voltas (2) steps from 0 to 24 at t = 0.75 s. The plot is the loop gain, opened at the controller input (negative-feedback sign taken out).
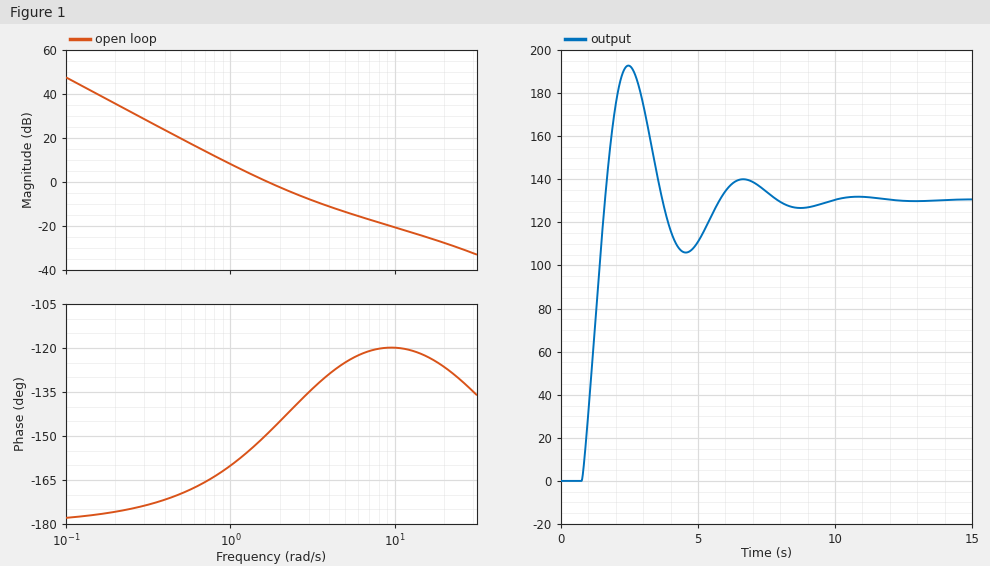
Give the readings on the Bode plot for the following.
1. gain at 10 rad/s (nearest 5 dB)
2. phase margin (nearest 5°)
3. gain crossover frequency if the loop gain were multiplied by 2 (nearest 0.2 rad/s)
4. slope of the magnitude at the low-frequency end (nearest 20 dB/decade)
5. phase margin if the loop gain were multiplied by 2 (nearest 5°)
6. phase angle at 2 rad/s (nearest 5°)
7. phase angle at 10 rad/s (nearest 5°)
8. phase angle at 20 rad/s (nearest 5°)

-20 dB
30°
2.6 rad/s
-40 dB/decade
40°
-145°
-120°
-125°
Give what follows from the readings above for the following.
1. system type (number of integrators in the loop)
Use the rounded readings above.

2
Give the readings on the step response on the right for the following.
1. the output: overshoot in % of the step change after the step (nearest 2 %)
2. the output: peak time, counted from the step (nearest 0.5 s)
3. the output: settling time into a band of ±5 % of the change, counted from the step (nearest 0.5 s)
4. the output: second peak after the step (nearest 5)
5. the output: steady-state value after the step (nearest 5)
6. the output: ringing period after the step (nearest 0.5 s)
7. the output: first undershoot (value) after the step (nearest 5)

48 %
1.5 s
6.5 s
140
130
4.0 s
105
